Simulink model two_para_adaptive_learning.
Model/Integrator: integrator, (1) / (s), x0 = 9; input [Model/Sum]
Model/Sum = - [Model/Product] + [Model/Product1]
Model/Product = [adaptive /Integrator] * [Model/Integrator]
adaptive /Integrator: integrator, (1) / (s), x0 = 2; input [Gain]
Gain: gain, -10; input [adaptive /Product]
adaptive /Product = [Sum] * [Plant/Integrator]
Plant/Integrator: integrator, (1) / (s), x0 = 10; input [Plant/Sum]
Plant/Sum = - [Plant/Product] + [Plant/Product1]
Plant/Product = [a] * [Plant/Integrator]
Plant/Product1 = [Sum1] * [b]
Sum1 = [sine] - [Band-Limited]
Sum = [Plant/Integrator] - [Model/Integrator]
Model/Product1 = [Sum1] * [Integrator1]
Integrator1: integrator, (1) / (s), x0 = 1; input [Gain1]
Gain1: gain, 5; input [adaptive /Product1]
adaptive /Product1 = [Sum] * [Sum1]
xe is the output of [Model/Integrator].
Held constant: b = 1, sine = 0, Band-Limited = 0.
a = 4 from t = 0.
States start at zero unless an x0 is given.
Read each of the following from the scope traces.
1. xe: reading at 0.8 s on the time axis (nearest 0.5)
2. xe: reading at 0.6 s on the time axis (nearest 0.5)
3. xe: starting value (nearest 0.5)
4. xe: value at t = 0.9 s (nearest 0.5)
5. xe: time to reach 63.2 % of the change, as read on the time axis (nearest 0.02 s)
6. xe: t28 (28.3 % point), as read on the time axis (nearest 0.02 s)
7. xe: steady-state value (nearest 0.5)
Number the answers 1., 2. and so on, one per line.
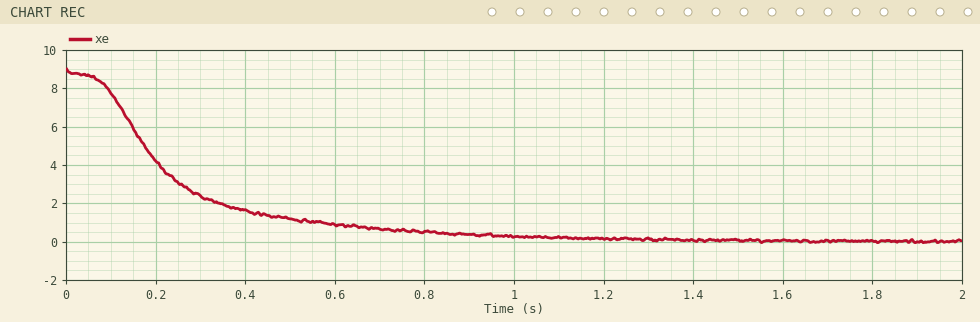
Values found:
1. 0.5
2. 1.0
3. 9.0
4. 0.5
5. 0.24 s
6. 0.14 s
7. 0.0
